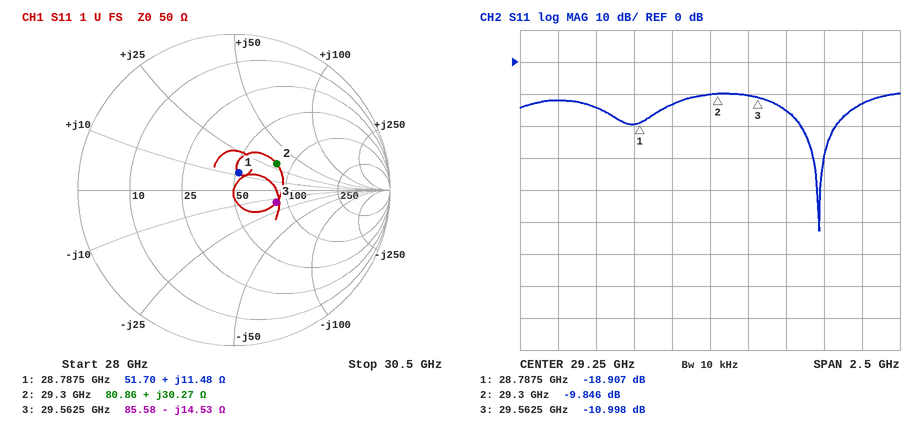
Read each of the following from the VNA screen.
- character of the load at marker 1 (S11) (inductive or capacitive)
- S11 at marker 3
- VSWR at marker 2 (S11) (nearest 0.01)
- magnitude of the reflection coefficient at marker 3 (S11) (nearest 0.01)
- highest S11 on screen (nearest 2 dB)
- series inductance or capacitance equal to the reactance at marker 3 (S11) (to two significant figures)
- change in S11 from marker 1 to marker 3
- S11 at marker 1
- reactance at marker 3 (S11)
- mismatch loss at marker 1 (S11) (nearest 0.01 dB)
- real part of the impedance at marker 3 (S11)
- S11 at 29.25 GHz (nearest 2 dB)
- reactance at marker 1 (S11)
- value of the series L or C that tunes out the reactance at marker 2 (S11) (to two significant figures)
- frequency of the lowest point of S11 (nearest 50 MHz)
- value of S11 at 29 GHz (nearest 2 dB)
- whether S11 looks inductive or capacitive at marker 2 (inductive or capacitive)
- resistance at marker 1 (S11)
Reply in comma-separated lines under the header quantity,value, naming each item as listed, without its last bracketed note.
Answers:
quantity,value
character of the load at marker 1 (S11),inductive
S11 at marker 3,-10.998 dB
VSWR at marker 2 (S11),1.95
magnitude of the reflection coefficient at marker 3 (S11),0.28
highest S11 on screen,-10 dB
series inductance or capacitance equal to the reactance at marker 3 (S11),370 fF
change in S11 from marker 1 to marker 3,7.909 dB
S11 at marker 1,-18.907 dB
reactance at marker 3,-14.53 Ω
mismatch loss at marker 1 (S11),0.06 dB
real part of the impedance at marker 3,85.58 Ω
S11 at 29.25 GHz,-10 dB
reactance at marker 1,+11.48 Ω
value of the series L or C that tunes out the reactance at marker 2 (S11),180 fF
frequency of the lowest point of S11,29.95 GHz
value of S11 at 29 GHz,-14 dB
whether S11 looks inductive or capacitive at marker 2,inductive
resistance at marker 1,51.70 Ω
